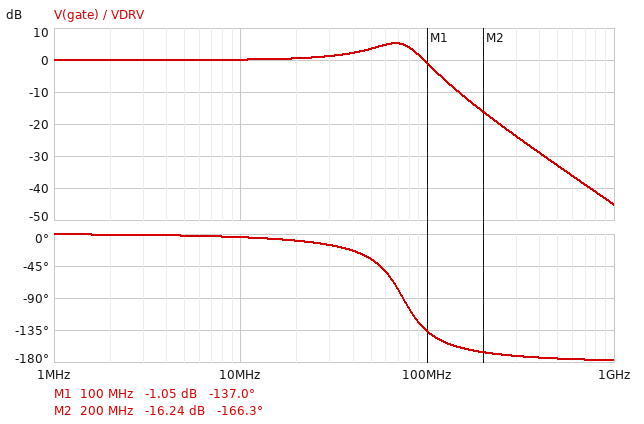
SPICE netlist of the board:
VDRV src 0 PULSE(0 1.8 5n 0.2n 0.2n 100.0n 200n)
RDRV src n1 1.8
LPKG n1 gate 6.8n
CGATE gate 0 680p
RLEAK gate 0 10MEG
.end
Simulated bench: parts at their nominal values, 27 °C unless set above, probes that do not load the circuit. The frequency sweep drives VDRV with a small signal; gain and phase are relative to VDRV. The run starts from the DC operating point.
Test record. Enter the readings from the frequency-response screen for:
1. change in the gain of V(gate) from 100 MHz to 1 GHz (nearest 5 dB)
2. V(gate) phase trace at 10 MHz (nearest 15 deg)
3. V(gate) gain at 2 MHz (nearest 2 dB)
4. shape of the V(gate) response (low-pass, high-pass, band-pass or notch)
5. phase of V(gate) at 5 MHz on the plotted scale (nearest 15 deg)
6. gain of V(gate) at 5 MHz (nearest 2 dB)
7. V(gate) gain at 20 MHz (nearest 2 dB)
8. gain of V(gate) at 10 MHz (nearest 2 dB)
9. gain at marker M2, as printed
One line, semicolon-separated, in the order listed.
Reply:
-45 dB; 0 deg; 0 dB; low-pass; 0 deg; 0 dB; 0 dB; 0 dB; -16.24 dB
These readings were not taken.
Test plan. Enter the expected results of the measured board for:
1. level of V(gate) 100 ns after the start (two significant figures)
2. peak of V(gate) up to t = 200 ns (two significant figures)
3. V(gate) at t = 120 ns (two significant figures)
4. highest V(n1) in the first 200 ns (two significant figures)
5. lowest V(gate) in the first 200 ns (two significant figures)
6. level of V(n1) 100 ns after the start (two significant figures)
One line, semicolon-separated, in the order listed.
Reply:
1.8 V; 2.5 V; 270 mV; 2.1 V; -710 mV; 1.8 V
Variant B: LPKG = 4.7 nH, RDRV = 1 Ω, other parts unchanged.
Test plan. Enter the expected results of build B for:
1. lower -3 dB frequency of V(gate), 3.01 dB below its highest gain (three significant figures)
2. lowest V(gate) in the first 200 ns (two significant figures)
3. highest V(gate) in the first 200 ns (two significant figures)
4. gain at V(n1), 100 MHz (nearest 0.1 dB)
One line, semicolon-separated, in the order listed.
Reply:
66.3 MHz; -980 mV; 2.8 V; -5.6 dB
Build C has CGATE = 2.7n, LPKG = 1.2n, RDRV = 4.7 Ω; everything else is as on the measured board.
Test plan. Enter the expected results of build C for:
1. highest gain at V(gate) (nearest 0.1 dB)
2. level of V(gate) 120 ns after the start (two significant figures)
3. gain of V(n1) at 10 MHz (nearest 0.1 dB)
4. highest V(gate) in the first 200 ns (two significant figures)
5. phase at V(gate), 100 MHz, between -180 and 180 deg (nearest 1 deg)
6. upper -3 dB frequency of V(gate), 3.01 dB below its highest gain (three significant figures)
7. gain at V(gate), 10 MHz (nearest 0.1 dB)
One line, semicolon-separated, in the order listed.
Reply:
0 dB; 560 mV; -2.2 dB; 1.8 V; -92 deg; 12.8 MHz; -2.1 dB
